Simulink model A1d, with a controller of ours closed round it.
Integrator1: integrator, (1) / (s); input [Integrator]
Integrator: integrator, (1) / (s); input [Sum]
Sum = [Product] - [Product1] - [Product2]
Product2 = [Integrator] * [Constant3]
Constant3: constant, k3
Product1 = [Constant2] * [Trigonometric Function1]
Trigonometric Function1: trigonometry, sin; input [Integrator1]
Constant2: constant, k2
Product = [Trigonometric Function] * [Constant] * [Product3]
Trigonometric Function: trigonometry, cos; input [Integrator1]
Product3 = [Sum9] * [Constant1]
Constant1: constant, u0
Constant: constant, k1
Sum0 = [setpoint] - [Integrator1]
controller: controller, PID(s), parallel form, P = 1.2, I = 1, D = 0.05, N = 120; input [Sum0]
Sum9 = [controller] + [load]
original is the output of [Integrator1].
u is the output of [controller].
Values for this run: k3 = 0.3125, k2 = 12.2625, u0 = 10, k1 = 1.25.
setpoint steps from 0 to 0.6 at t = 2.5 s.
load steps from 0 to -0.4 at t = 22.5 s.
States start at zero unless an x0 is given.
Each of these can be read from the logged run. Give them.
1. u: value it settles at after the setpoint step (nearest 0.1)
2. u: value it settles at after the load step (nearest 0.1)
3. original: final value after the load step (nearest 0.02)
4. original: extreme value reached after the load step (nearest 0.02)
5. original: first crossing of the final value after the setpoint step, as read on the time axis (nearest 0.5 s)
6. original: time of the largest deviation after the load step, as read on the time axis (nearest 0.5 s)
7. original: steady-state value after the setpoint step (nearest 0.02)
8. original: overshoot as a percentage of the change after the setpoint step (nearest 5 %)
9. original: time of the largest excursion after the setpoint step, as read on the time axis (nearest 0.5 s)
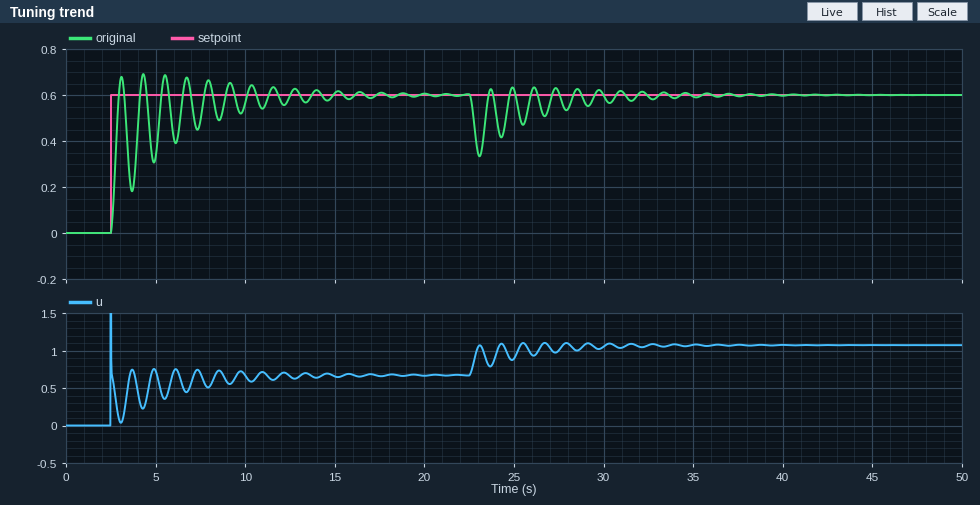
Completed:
0.7
1.1
0.60
0.34
3.0 s
23.0 s
0.60
15 %
4.5 s
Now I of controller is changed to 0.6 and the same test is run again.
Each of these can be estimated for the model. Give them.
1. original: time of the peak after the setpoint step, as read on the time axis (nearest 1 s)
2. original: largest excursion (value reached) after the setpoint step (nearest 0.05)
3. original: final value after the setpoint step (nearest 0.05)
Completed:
3 s
0.65
0.60
